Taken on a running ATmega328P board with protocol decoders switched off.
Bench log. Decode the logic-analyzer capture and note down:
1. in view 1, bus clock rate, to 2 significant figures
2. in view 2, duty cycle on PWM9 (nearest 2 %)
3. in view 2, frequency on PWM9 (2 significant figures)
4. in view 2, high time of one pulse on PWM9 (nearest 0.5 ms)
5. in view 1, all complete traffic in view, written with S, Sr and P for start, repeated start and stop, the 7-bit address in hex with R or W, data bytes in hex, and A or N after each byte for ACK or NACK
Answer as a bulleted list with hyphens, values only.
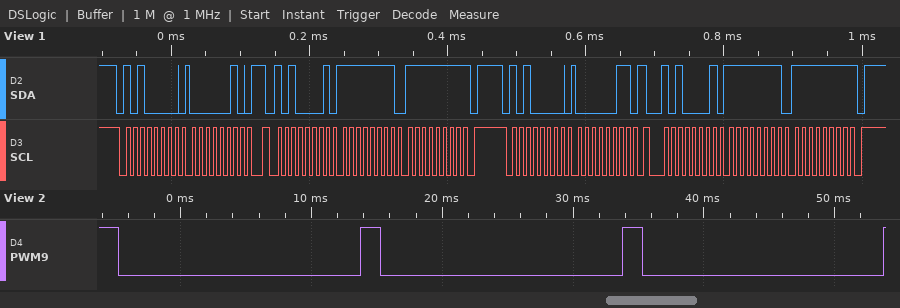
- 100 kHz
- 8 %
- 50 Hz
- 1.5 ms
- S 50W A 02 A Sr 50R A FF A FF N P S 50W A 03 A Sr 50R A FF A FF N P
